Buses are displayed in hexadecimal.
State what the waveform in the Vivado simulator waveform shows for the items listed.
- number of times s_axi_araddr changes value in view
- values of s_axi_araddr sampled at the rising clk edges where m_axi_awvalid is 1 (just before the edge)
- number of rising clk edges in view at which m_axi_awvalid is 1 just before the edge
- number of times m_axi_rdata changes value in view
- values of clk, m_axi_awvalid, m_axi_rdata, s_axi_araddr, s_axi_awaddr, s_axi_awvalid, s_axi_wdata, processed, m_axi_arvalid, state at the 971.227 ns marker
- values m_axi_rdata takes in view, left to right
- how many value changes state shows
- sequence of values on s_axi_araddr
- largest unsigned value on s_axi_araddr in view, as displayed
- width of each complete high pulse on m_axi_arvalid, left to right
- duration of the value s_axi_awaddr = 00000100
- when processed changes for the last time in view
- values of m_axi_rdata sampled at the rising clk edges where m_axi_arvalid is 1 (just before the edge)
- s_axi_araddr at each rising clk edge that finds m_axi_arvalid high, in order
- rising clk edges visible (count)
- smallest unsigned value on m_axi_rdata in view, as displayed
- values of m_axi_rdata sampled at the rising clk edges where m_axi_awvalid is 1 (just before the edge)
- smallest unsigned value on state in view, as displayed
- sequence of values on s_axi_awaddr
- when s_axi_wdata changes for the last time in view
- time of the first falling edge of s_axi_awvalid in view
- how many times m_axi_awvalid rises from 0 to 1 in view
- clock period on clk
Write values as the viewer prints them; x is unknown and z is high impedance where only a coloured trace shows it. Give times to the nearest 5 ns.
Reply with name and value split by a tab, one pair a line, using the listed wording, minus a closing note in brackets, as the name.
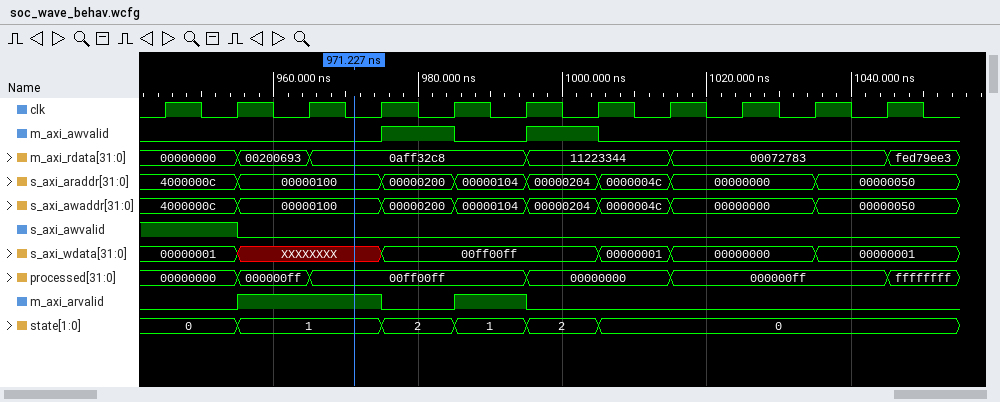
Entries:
number of times s_axi_araddr changes value in view	7
values of s_axi_araddr sampled at the rising clk edges where m_axi_awvalid is 1	00000200, 00000204
number of rising clk edges in view at which m_axi_awvalid is 1 just before the edge	2
number of times m_axi_rdata changes value in view	5
values of clk, m_axi_awvalid, m_axi_rdata, s_axi_araddr, s_axi_awaddr, s_axi_awvalid, s_axi_wdata, processed, m_axi_arvalid, state at the 971.227 ns marker	clk=0, m_axi_awvalid=0, m_axi_rdata=0aff32c8, s_axi_araddr=00000100, s_axi_awaddr=00000100, s_axi_awvalid=0, s_axi_wdata=XXXXXXXX, processed=00ff00ff, m_axi_arvalid=1, state=1
values m_axi_rdata takes in view, left to right	00000000, 00200693, 0aff32c8, 11223344, 00072783, fed79ee3
how many value changes state shows	5
sequence of values on s_axi_araddr	4000000c, 00000100, 00000200, 00000104, 00000204, 0000004c, 00000000, 00000050
largest unsigned value on s_axi_araddr in view, as displayed	4000000c
width of each complete high pulse on m_axi_arvalid, left to right	20 ns, 10 ns
duration of the value s_axi_awaddr = 00000100	20 ns
when processed changes for the last time in view	1045 ns
values of m_axi_rdata sampled at the rising clk edges where m_axi_arvalid is 1	00200693, 0aff32c8, 0aff32c8
s_axi_araddr at each rising clk edge that finds m_axi_arvalid high, in order	00000100, 00000100, 00000104
rising clk edges visible	11
smallest unsigned value on m_axi_rdata in view, as displayed	00000000
values of m_axi_rdata sampled at the rising clk edges where m_axi_awvalid is 1	0aff32c8, 11223344
smallest unsigned value on state in view, as displayed	0
sequence of values on s_axi_awaddr	4000000c, 00000100, 00000200, 00000104, 00000204, 0000004c, 00000000, 00000050
when s_axi_wdata changes for the last time in view	1035 ns
time of the first falling edge of s_axi_awvalid in view	955 ns
how many times m_axi_awvalid rises from 0 to 1 in view	2
clock period on clk	10 ns
